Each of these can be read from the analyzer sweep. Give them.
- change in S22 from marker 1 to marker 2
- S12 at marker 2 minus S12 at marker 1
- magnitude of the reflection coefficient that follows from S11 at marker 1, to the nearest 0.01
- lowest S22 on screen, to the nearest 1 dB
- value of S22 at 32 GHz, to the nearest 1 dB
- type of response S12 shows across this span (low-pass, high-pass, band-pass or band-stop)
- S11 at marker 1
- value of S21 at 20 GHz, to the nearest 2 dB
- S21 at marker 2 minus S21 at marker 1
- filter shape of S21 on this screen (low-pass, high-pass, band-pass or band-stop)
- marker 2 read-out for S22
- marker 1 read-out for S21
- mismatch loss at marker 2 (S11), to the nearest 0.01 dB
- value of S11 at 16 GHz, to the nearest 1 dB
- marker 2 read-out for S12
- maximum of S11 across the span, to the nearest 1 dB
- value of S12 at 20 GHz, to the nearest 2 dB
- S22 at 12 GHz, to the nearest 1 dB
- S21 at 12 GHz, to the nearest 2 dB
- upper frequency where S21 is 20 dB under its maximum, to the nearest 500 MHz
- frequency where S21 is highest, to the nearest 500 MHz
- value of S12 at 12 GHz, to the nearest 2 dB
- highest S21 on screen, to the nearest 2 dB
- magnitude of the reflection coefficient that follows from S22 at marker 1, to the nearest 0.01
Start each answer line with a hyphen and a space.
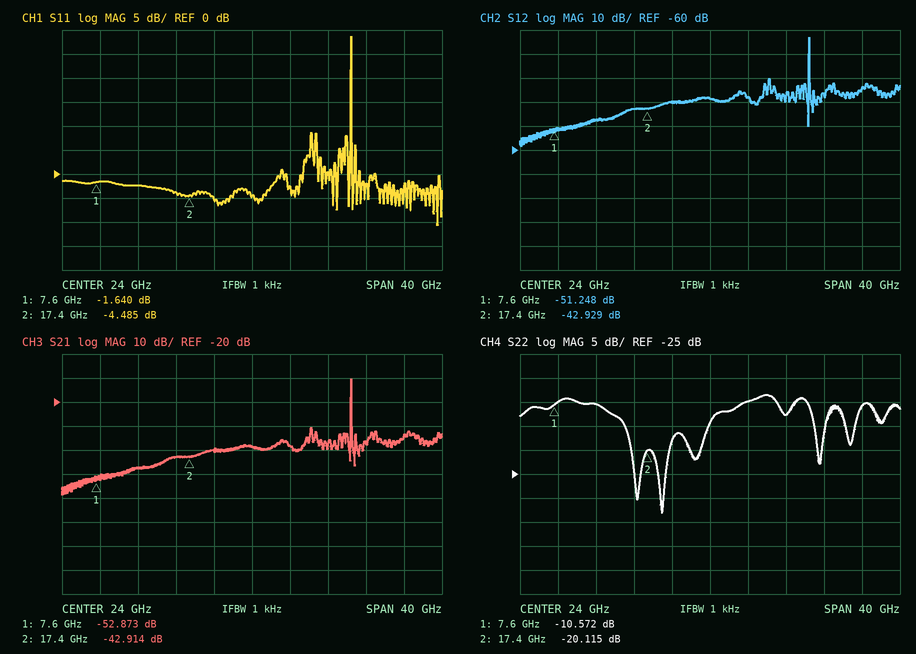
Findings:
- -9.543 dB
- 8.319 dB
- 0.83
- -33 dB
- -13 dB
- band-pass
- -1.640 dB
- -40 dB
- 9.959 dB
- band-pass
- -20.115 dB
- -52.873 dB
- 1.91 dB
- -4 dB
- -42.929 dB
- 29 dB
- -40 dB
- -10 dB
- -48 dB
- 34.5 GHz
- 34.5 GHz
- -48 dB
- -10 dB
- 0.30
